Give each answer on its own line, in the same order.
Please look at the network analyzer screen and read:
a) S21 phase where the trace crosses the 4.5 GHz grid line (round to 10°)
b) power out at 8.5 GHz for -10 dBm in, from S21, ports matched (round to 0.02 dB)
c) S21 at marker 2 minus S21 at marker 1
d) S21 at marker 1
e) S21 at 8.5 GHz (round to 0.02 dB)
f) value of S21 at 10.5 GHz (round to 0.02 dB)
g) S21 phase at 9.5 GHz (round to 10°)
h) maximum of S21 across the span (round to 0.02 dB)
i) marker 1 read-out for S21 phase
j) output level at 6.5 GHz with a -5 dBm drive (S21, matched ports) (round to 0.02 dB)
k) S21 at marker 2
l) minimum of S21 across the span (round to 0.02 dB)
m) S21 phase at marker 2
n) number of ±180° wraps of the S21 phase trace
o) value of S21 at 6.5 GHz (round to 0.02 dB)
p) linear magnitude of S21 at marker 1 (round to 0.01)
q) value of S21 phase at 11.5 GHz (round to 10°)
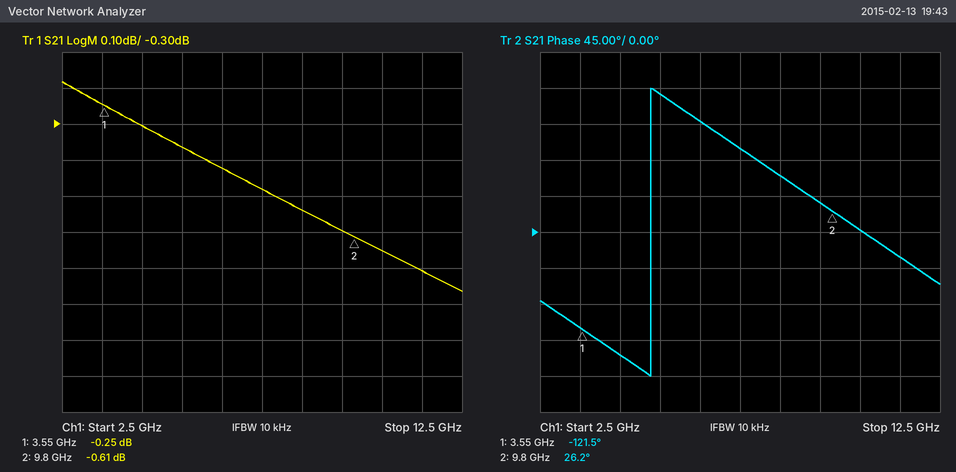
-150°
-10.54 dBm
-0.36 dB
-0.25 dB
-0.54 dB
-0.66 dB
40°
-0.18 dB
-121.5°
-5.42 dBm
-0.61 dB
-0.76 dB
26.2°
1
-0.42 dB
0.97
-30°
